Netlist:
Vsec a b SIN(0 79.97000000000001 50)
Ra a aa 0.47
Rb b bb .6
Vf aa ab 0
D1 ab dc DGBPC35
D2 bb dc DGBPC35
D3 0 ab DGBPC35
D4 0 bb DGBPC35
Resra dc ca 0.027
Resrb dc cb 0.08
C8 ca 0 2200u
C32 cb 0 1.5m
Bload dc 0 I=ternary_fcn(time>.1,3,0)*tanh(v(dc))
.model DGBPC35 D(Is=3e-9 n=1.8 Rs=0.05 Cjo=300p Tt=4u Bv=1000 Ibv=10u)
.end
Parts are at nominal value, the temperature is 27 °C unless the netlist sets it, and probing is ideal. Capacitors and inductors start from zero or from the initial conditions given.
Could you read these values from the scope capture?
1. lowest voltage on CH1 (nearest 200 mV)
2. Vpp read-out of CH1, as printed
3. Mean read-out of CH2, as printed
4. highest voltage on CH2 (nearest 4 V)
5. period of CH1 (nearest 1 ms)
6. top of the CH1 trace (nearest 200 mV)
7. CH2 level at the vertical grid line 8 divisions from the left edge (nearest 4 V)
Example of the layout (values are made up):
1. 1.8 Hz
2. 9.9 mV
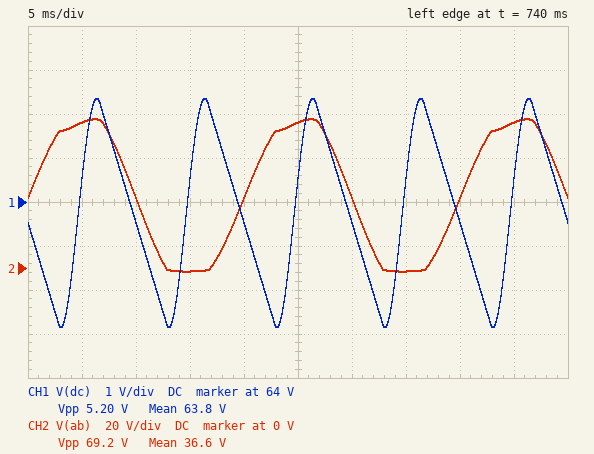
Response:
1. 61.2 V
2. 5.20 V
3. 36.6 V
4. 68 V
5. 10 ms
6. 66.4 V
7. 32 V
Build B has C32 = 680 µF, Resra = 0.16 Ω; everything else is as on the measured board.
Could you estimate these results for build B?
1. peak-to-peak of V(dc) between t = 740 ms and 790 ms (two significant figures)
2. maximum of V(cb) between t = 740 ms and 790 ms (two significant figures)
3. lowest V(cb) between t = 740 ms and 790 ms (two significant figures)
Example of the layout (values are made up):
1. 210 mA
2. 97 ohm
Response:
1. 6.9 V
2. 67 V
3. 60 V
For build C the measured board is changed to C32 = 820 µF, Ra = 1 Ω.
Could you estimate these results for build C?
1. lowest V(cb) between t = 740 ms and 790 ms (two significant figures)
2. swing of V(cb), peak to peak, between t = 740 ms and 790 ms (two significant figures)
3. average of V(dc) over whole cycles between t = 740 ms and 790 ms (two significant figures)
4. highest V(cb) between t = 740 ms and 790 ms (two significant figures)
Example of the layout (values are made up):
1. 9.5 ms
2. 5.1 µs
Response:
1. 57 V
2. 5.9 V
3. 60 V
4. 63 V
